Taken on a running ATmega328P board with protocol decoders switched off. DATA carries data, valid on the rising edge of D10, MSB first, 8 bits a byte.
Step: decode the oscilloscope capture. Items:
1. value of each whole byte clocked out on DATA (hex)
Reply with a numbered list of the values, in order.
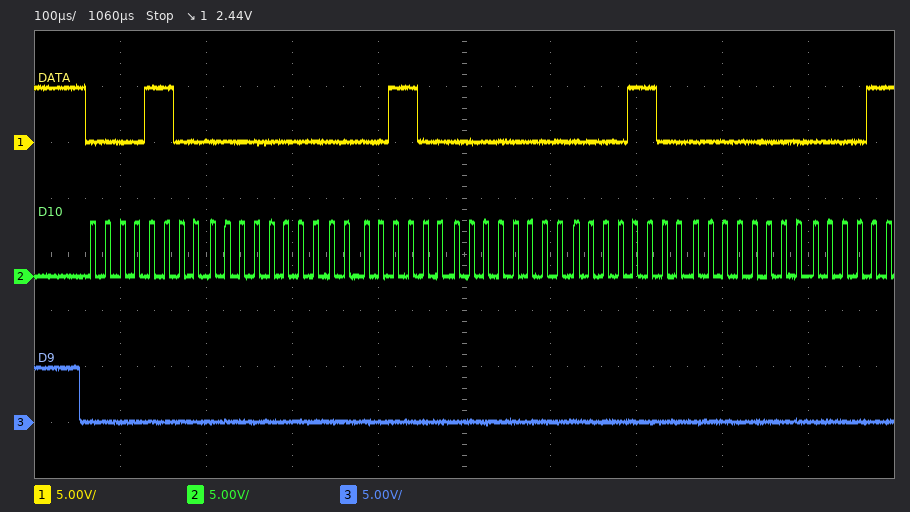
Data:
1. 0C 00 0C 00 0C 00
